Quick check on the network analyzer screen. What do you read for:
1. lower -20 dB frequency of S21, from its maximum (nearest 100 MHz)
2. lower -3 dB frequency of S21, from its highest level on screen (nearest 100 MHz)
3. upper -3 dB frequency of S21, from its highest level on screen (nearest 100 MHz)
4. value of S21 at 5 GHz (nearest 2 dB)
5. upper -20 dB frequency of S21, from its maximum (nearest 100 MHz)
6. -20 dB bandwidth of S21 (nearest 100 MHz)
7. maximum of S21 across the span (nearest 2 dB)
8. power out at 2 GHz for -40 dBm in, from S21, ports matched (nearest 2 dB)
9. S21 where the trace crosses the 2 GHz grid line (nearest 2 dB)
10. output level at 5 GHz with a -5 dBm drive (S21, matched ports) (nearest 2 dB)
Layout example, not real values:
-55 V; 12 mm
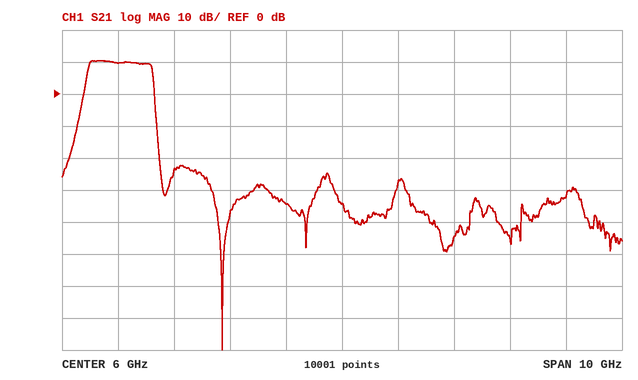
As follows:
1.3 GHz; 1.5 GHz; 2.6 GHz; -34 dB; 2.7 GHz; 1.4 GHz; 10 dB; -30 dBm; 10 dB; -40 dBm
